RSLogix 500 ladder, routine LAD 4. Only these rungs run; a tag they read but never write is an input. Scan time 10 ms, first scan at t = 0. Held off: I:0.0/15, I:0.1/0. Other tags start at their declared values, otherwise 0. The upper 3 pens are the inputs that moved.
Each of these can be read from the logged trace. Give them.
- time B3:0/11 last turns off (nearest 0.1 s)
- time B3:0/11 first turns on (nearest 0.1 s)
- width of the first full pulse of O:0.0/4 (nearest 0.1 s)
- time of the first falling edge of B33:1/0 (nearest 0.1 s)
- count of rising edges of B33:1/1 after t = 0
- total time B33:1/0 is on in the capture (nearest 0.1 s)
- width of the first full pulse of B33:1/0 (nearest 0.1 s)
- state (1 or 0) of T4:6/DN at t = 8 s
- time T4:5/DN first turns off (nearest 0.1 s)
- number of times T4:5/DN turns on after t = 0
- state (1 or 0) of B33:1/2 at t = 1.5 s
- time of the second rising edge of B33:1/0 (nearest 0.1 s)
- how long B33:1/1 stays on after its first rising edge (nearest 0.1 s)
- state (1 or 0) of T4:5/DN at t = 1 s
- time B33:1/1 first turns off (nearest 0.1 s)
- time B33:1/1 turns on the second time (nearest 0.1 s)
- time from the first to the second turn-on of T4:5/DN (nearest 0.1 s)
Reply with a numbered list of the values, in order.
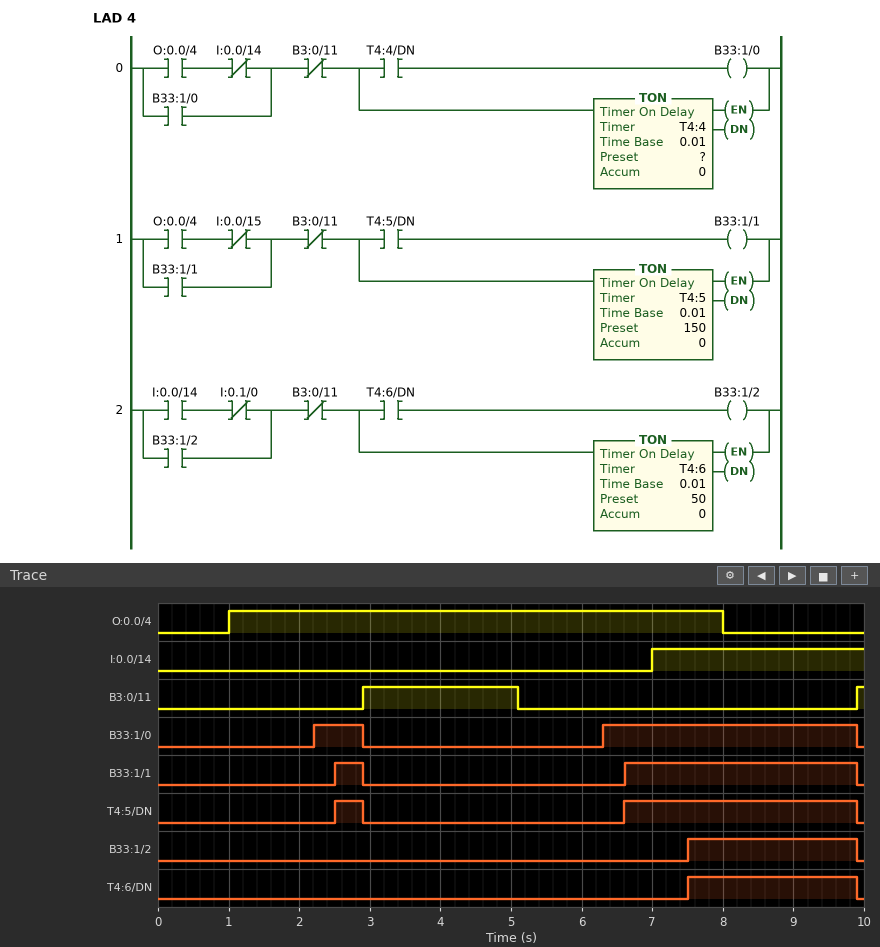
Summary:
1. 5.1 s
2. 2.9 s
3. 7.0 s
4. 2.9 s
5. 2
6. 4.3 s
7. 0.7 s
8. 1
9. 2.9 s
10. 2
11. 0
12. 6.3 s
13. 0.4 s
14. 0
15. 2.9 s
16. 6.6 s
17. 4.1 s
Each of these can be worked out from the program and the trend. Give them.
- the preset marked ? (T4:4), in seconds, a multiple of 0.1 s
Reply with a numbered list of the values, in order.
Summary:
1. 1.2 s
